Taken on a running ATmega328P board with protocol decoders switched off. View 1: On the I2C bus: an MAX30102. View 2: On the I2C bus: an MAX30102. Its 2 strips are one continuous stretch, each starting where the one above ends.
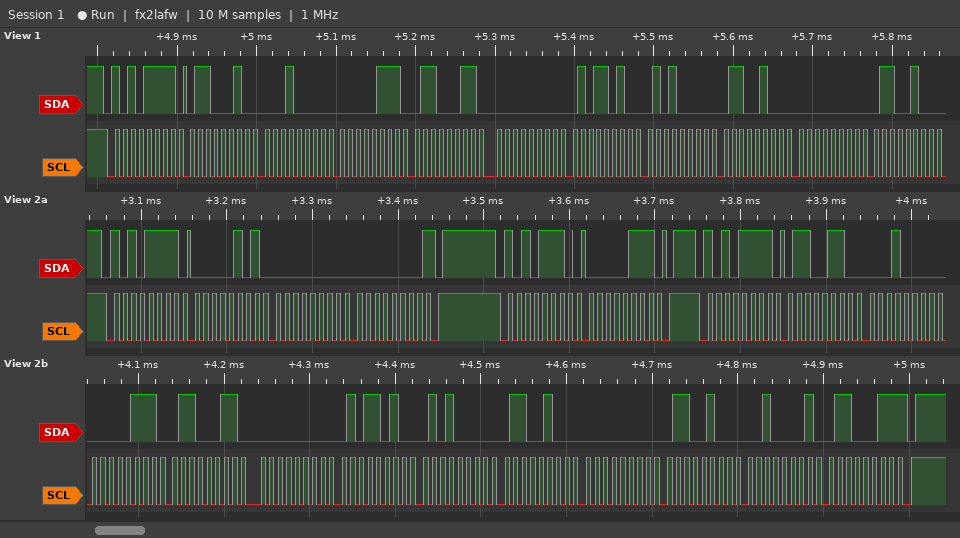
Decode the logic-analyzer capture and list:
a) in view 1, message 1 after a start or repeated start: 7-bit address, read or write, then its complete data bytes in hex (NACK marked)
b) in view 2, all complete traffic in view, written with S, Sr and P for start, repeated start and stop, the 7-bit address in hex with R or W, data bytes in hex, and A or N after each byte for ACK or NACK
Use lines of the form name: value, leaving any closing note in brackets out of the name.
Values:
in view 1, message 1 after a start or repeated start: 7-bit address, read or write, then its complete data bytes in hex: 0x57 read: 62 10 07 63 00 5A 50 64 00 64
in view 2, all complete traffic in view, written with S, Sr and P for start, repeated start and stop, the 7-bit address in hex with R or W, data bytes in hex, and A or N after each byte for ACK or NACK: S 57R A 05 A 00 A 00 N P S 57W A 07 A P S 57R A 66 A 10 A 07 A 63 A 00 A 5A A 50 A 64 A 00 A 64 A 21 A 63 N P
